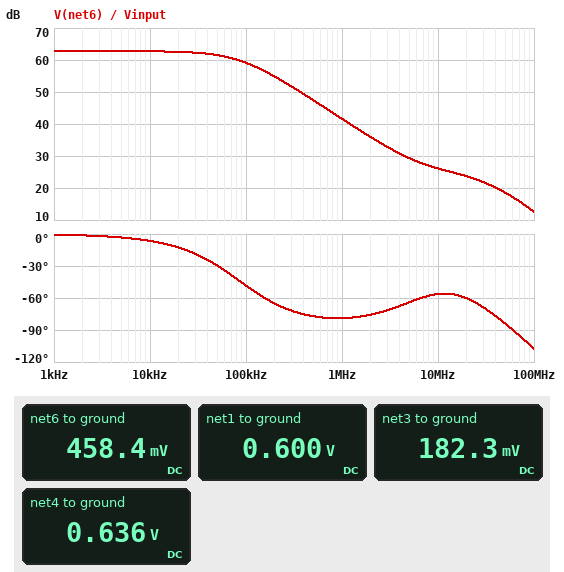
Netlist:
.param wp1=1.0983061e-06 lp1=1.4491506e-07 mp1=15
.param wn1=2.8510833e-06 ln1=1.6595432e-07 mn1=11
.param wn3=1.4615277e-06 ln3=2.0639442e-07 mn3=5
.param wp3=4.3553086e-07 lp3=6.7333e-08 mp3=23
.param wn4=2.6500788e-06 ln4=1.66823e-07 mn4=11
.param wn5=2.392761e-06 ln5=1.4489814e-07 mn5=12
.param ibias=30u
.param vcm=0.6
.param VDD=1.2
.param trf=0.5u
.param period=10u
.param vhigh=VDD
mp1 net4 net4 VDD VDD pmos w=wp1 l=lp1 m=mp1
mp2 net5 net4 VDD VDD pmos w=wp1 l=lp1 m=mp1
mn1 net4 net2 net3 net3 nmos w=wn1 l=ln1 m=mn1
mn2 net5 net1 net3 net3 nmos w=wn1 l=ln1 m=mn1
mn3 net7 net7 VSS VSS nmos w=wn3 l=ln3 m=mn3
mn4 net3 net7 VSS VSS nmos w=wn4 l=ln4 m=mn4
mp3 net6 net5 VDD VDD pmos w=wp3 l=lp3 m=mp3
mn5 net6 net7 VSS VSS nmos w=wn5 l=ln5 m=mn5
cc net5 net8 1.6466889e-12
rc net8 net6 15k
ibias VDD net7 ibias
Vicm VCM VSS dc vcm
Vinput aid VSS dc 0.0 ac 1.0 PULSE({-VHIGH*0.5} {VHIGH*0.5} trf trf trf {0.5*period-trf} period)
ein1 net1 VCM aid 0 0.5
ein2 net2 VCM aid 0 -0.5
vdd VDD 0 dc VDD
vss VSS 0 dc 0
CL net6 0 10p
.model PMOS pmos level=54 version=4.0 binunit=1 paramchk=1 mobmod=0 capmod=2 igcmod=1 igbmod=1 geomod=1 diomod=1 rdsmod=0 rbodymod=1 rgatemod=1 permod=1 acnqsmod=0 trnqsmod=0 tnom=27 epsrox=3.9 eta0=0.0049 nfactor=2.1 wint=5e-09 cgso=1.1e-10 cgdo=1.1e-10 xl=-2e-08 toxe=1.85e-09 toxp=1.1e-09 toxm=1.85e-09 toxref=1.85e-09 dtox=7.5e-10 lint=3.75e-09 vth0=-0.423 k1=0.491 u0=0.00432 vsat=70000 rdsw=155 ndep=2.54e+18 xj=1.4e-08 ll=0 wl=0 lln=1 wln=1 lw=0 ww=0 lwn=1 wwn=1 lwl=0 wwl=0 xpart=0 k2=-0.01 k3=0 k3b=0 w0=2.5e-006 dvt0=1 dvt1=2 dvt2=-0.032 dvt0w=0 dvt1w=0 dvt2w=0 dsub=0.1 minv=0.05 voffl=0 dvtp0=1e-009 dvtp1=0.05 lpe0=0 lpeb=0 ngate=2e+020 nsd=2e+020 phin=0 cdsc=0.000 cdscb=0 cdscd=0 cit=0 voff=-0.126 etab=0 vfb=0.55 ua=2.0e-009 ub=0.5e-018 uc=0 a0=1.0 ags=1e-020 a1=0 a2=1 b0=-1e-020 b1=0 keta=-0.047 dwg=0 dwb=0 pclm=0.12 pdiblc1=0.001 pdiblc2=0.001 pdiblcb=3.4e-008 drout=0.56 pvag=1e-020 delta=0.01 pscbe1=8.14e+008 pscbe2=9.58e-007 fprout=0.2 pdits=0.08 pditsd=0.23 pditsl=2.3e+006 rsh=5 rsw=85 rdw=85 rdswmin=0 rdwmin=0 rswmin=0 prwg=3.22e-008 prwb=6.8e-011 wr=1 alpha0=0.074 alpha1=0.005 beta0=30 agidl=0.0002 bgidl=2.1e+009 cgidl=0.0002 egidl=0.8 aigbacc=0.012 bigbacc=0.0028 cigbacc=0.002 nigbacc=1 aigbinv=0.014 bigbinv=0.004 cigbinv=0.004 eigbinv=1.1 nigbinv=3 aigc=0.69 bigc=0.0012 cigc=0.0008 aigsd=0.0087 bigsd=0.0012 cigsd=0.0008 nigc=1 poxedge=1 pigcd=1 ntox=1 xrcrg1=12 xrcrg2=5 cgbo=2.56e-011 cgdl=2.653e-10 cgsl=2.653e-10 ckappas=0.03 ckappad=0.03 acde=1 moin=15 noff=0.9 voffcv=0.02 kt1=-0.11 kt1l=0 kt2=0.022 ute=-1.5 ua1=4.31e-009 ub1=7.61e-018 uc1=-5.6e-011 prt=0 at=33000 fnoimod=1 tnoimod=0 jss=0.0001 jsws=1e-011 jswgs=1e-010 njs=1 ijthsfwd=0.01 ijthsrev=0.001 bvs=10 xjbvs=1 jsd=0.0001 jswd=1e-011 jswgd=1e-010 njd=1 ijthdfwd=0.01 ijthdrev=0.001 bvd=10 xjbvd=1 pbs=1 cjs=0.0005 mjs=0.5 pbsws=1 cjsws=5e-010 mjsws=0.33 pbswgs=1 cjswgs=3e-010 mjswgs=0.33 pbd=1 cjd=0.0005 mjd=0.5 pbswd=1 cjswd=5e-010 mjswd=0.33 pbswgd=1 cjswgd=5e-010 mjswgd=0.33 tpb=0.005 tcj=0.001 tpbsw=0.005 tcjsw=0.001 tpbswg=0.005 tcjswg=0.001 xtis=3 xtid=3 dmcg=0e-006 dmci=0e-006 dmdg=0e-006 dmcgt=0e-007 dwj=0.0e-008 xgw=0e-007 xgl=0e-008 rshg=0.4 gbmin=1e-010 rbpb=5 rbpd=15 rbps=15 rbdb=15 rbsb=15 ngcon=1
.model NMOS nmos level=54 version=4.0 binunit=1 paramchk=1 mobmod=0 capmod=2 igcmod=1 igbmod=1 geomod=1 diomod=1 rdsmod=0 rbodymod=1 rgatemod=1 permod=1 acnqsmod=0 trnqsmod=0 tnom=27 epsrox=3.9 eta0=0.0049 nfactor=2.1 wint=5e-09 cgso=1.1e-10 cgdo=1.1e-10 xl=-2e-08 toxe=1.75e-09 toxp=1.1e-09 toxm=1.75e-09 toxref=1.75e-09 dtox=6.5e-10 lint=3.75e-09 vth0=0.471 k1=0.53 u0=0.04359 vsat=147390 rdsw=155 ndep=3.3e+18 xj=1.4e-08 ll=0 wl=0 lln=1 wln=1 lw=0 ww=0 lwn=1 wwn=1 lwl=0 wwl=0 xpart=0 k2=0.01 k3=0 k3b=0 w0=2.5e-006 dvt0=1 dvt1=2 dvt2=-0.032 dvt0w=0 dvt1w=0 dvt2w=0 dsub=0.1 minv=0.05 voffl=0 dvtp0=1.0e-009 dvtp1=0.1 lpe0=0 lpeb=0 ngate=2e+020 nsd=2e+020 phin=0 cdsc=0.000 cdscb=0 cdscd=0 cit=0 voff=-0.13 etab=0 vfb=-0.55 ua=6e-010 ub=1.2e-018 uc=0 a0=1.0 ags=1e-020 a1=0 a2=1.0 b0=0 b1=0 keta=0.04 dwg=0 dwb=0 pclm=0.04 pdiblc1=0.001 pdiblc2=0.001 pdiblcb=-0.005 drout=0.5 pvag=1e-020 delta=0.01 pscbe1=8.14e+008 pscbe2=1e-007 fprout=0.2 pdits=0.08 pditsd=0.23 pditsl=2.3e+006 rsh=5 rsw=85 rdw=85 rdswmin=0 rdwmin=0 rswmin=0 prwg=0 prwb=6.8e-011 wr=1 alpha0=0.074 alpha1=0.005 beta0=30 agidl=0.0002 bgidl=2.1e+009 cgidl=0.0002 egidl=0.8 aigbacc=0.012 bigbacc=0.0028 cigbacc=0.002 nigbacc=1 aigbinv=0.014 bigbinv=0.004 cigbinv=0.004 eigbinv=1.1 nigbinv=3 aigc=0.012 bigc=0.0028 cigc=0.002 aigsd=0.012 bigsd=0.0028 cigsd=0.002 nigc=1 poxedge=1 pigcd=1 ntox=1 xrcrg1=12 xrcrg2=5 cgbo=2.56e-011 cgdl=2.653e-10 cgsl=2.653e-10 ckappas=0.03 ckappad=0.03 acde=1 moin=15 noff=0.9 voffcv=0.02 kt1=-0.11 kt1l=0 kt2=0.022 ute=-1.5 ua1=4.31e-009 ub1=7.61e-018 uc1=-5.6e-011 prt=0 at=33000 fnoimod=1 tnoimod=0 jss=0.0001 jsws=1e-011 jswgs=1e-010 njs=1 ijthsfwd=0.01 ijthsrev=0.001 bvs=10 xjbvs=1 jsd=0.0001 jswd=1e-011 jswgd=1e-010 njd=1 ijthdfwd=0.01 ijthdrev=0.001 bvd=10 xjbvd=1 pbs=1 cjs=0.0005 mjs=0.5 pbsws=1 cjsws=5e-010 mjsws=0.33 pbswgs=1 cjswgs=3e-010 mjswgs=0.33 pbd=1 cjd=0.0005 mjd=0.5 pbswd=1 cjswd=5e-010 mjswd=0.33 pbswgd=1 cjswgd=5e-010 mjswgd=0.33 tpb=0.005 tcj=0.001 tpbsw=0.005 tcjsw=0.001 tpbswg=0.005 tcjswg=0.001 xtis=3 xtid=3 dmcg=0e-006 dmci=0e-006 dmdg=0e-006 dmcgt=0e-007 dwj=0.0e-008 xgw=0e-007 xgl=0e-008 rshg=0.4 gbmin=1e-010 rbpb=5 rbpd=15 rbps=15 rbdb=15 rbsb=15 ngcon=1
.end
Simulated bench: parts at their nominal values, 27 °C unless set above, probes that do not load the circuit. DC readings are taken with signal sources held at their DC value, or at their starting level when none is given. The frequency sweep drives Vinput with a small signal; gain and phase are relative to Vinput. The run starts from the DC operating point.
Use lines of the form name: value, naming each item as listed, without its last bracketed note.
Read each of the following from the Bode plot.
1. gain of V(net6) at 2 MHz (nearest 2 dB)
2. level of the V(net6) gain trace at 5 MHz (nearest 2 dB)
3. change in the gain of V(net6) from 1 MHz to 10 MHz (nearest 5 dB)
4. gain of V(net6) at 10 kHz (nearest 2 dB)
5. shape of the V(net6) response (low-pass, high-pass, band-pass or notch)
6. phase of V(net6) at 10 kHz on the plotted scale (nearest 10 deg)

gain of V(net6) at 2 MHz: 36 dB
level of the V(net6) gain trace at 5 MHz: 30 dB
change in the gain of V(net6) from 1 MHz to 10 MHz: -15 dB
gain of V(net6) at 10 kHz: 62 dB
shape of the V(net6) response: low-pass
phase of V(net6) at 10 kHz on the plotted scale: -10 deg
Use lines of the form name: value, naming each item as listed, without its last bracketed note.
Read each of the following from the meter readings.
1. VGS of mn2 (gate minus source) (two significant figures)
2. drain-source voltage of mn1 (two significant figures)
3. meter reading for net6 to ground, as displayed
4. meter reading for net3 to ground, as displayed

VGS of mn2 (gate minus source): 420 mV
drain-source voltage of mn1: 450 mV
meter reading for net6 to ground, as displayed: 458.4 mV
meter reading for net3 to ground, as displayed: 182.3 mV
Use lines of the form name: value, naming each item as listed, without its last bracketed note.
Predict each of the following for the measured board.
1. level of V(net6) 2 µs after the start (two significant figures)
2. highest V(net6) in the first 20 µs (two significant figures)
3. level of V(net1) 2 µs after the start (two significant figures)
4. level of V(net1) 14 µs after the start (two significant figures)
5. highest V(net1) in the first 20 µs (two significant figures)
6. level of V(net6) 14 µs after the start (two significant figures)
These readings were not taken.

level of V(net6) 2 µs after the start: 1.2 V
highest V(net6) in the first 20 µs: 1.2 V
level of V(net1) 2 µs after the start: 900 mV
level of V(net1) 14 µs after the start: 900 mV
highest V(net1) in the first 20 µs: 900 mV
level of V(net6) 14 µs after the start: 1.2 V
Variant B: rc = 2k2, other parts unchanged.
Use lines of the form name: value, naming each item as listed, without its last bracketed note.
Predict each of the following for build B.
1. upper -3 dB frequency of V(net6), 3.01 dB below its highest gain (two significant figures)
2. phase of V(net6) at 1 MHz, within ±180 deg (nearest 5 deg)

upper -3 dB frequency of V(net6), 3.01 dB below its highest gain: 88 kHz
phase of V(net6) at 1 MHz, within ±180 deg: -85 deg
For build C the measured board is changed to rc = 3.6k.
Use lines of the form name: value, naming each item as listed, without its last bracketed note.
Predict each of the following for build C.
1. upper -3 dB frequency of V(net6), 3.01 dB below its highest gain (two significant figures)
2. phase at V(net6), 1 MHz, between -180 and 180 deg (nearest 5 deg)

upper -3 dB frequency of V(net6), 3.01 dB below its highest gain: 88 kHz
phase at V(net6), 1 MHz, between -180 and 180 deg: -85 deg
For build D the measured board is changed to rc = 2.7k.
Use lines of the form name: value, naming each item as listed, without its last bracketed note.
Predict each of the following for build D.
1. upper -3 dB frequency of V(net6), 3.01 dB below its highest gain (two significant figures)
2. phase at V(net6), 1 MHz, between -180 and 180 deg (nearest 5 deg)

upper -3 dB frequency of V(net6), 3.01 dB below its highest gain: 88 kHz
phase at V(net6), 1 MHz, between -180 and 180 deg: -85 deg
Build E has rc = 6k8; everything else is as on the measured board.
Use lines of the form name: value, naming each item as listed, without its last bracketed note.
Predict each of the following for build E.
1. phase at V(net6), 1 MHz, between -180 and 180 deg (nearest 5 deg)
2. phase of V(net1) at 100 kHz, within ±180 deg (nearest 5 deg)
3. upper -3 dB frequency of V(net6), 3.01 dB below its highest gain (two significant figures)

phase at V(net6), 1 MHz, between -180 and 180 deg: -85 deg
phase of V(net1) at 100 kHz, within ±180 deg: 0 deg
upper -3 dB frequency of V(net6), 3.01 dB below its highest gain: 88 kHz
